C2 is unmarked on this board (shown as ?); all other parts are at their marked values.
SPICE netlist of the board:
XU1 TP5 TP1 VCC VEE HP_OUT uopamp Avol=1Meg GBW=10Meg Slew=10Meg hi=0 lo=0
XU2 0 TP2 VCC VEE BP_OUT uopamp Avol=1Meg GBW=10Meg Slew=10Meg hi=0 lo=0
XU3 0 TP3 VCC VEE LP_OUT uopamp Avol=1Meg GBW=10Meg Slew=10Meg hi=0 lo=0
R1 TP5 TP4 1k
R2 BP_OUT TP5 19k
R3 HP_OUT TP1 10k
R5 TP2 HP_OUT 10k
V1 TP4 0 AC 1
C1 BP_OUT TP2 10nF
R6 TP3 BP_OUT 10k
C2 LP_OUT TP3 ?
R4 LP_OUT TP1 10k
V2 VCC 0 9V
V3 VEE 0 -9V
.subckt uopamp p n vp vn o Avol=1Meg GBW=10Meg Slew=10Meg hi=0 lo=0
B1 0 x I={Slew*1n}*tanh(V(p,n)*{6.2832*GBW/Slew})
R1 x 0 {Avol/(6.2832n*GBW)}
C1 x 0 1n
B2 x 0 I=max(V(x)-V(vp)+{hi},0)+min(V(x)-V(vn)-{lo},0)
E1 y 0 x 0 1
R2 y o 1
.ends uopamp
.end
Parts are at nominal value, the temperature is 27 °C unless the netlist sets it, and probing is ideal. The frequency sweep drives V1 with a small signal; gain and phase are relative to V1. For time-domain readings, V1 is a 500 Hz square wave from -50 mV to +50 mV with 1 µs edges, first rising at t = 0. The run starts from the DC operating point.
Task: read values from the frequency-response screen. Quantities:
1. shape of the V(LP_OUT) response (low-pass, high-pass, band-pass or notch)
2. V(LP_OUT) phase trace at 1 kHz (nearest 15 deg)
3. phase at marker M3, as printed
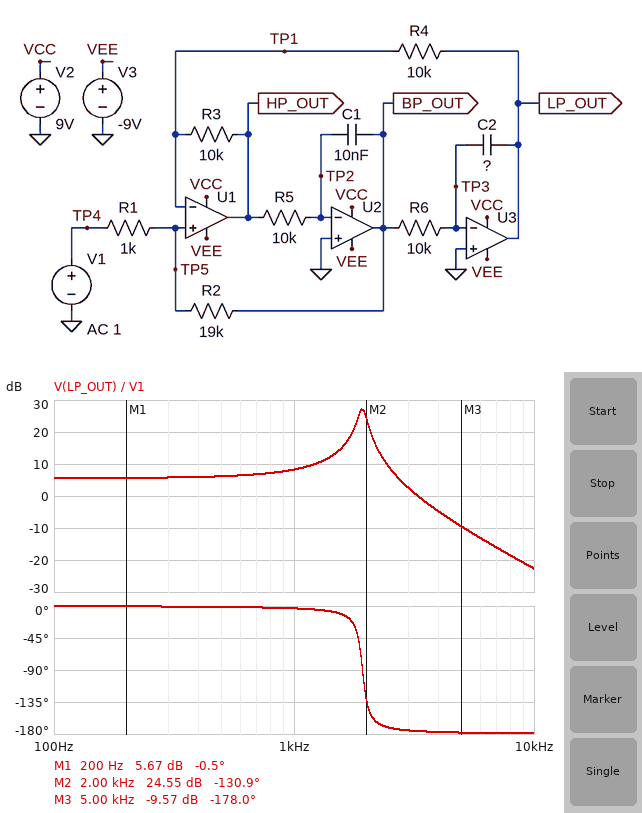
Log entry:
low-pass
0 deg
-178.0 deg
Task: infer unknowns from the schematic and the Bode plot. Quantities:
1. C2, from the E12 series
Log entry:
6.8 nF
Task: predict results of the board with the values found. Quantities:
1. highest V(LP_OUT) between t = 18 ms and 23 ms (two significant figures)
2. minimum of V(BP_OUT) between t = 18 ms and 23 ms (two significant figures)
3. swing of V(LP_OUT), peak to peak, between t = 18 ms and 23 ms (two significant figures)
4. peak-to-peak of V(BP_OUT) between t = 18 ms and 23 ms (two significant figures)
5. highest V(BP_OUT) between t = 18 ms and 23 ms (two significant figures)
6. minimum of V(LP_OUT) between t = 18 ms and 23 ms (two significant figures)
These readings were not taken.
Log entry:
200 mV
-94 mV
400 mV
190 mV
94 mV
-200 mV
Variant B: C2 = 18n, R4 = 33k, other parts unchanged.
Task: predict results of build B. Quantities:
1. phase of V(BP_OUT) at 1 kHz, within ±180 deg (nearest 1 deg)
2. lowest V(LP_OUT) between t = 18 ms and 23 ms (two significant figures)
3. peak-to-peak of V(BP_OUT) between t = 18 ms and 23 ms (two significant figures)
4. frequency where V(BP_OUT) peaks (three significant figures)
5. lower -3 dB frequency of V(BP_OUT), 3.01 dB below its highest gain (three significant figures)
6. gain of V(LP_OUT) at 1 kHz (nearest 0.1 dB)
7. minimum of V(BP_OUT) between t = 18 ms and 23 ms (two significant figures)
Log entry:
100 deg
-620 mV
690 mV
653 Hz
603 Hz
9.5 dB
-350 mV
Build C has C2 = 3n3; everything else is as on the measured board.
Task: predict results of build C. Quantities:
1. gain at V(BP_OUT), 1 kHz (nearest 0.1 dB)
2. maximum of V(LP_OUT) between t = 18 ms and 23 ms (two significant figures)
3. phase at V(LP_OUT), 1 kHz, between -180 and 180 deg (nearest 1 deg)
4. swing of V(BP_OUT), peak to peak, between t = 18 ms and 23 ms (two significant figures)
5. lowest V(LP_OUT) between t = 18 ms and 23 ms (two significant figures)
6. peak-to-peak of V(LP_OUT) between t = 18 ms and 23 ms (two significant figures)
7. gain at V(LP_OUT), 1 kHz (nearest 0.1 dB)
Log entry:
-6.9 dB
240 mV
-1 deg
170 mV
-240 mV
480 mV
6.8 dB
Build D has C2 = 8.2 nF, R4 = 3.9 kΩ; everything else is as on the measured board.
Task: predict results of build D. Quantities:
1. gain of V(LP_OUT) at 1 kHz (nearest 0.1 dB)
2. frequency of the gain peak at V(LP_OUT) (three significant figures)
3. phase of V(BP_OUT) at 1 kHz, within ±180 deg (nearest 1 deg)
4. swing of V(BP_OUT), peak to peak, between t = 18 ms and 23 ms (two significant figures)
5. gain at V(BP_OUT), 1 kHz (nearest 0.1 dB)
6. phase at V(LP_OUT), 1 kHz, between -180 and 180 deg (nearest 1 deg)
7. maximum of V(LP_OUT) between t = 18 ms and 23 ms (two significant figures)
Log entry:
3.6 dB
2.81 kHz
-92 deg
300 mV
-2.2 dB
-2 deg
160 mV
